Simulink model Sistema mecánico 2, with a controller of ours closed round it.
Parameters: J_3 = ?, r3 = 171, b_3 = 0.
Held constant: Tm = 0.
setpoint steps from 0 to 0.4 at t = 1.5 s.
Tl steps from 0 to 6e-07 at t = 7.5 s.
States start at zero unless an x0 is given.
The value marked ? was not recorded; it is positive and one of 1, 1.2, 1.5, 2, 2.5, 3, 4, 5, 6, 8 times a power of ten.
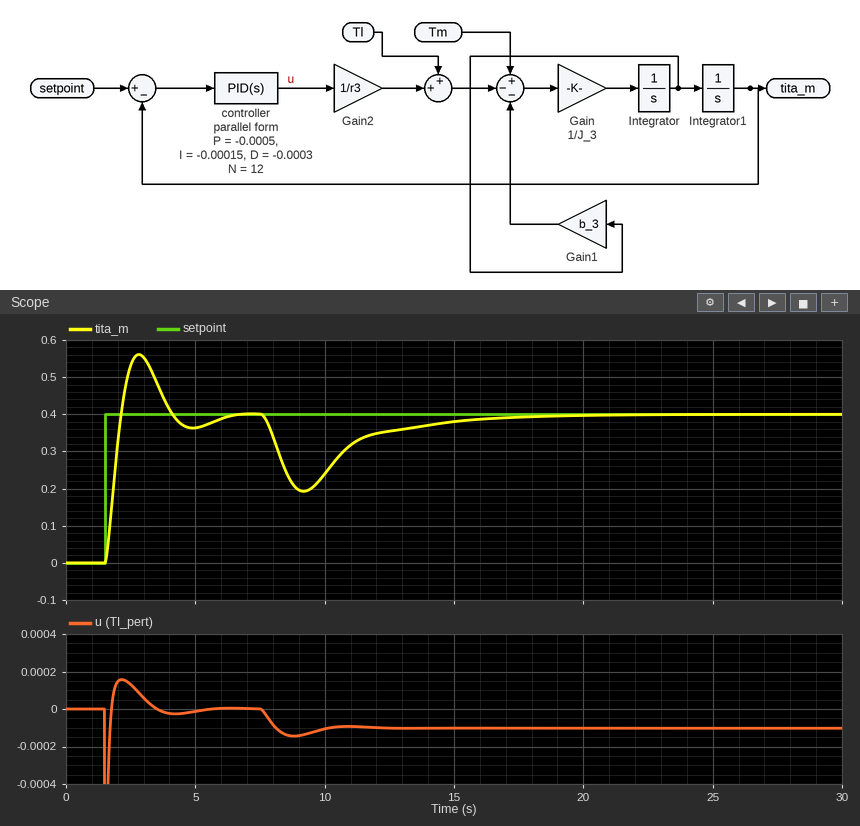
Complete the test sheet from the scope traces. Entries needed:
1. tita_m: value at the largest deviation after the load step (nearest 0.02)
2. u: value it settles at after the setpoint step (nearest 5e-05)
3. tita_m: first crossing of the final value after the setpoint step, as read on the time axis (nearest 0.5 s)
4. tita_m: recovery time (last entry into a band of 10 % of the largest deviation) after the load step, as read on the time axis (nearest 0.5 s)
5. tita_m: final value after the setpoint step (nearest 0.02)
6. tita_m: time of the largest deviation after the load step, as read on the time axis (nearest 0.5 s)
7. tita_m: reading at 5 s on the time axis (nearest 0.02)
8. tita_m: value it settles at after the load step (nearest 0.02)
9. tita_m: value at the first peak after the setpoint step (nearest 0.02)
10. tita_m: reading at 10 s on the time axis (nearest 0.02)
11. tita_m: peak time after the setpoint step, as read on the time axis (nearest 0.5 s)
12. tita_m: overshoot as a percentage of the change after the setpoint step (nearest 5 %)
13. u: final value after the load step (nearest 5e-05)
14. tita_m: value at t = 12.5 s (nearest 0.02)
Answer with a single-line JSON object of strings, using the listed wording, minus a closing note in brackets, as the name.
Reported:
{"tita_m: value at the largest deviation after the load step": "0.20", "u: value it settles at after the setpoint step": "0.00000", "tita_m: first crossing of the final value after the setpoint step, as read on the time axis": "2.0 s", "tita_m: recovery time (last entry into a band of 10 % of the largest deviation) after the load step, as read on the time axis": "15.0 s", "tita_m: final value after the setpoint step": "0.40", "tita_m: time of the largest deviation after the load step, as read on the time axis": "9.0 s", "tita_m: reading at 5 s on the time axis": "0.36", "tita_m: value it settles at after the load step": "0.40", "tita_m: value at the first peak after the setpoint step": "0.56", "tita_m: reading at 10 s on the time axis": "0.24", "tita_m: peak time after the setpoint step, as read on the time axis": "3.0 s", "tita_m: overshoot as a percentage of the change after the setpoint step": "40 %", "u: final value after the load step": "-0.00010", "tita_m: value at t = 12.5 s": "0.36"}
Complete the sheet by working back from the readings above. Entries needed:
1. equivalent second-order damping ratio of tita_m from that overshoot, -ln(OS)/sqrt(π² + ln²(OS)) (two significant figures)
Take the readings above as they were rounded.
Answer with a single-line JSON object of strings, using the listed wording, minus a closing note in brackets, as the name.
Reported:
{"equivalent second-order damping ratio of tita_m from that overshoot, -ln(OS)/sqrt(π² + ln²(OS))": "0.28"}
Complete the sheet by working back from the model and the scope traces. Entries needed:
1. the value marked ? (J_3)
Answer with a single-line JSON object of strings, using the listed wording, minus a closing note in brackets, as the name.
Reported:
{"the value marked ?": "1e-06"}
